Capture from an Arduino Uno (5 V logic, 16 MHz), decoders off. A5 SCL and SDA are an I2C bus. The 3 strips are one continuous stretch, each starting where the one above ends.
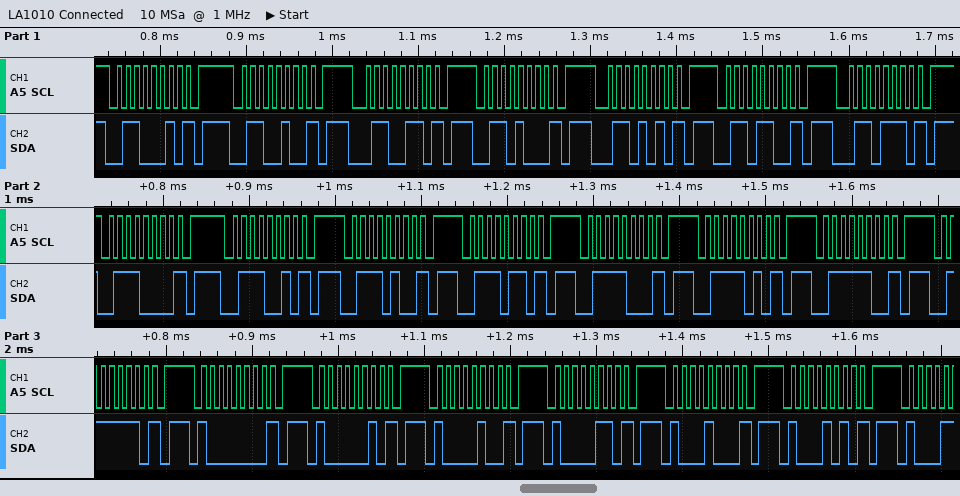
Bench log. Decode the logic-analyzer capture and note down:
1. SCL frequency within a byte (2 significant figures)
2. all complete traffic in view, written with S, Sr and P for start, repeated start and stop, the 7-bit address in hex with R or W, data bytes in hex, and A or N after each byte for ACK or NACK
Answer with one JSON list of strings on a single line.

["100 kHz", "S 31W N P S 32W N P S 33W N P S 34W N P S 35W N P S 36W N P S 37W N P S 38W N P S 39W N P S 3AW N P S 3BW N P S 3CW N P S 3DW N P S 3EW N P S 3FW N P S 40W N P S 41W N P S 42W N P S 43W N P S 44W N P S 45W N P"]
